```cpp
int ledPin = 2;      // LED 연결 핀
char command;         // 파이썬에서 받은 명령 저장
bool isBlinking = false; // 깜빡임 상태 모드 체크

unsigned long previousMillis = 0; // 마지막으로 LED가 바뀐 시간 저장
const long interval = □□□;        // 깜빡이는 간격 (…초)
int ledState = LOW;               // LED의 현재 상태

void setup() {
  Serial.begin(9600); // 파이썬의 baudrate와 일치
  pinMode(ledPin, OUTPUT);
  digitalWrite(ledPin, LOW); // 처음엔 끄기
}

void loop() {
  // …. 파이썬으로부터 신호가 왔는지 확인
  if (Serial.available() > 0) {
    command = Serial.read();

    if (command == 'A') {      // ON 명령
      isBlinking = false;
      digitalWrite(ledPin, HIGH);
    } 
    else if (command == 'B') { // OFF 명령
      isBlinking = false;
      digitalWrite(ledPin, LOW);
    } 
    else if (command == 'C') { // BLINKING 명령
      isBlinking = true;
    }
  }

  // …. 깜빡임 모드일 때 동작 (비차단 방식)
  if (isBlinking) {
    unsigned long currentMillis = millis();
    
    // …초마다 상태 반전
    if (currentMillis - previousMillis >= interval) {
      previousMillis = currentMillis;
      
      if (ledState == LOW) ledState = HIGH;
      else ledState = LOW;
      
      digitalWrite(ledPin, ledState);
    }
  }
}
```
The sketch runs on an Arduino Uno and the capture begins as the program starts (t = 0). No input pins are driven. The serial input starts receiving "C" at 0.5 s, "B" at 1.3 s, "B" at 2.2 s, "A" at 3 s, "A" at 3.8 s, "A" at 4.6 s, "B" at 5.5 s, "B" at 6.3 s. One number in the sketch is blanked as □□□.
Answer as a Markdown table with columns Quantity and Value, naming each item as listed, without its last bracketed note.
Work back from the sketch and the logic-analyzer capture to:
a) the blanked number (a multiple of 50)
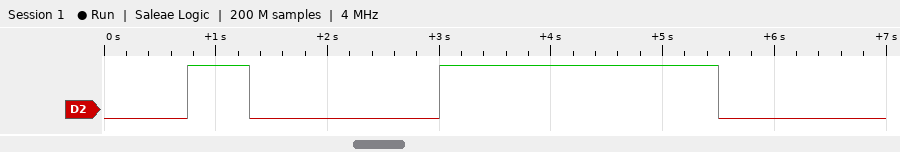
| Quantity | Value |
|---|---|
| the blanked number | 750 |
